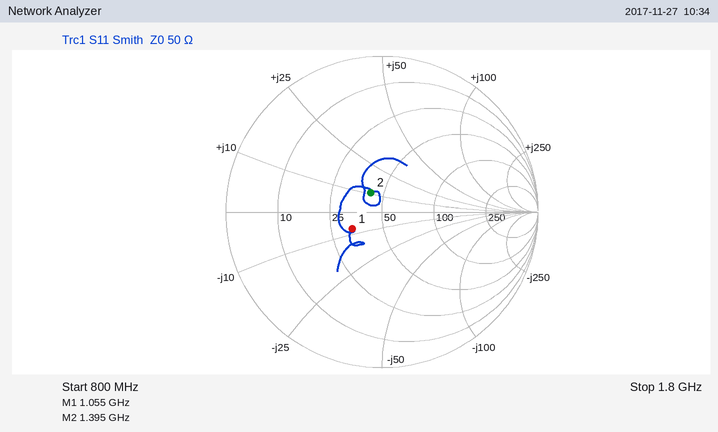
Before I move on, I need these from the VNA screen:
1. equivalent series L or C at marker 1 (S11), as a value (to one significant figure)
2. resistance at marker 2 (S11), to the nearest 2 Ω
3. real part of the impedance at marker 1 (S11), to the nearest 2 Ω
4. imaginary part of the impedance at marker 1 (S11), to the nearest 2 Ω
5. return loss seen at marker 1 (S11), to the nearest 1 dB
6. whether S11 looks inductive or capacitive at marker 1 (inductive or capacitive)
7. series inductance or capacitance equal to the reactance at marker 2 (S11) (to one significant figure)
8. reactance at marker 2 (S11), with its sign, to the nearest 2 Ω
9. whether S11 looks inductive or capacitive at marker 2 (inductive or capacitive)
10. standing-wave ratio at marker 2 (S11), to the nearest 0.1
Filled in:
20 pF
42 Ω
34 Ω
-8 Ω
13 dB
capacitive
1 nH
+10 Ω
inductive
1.3
